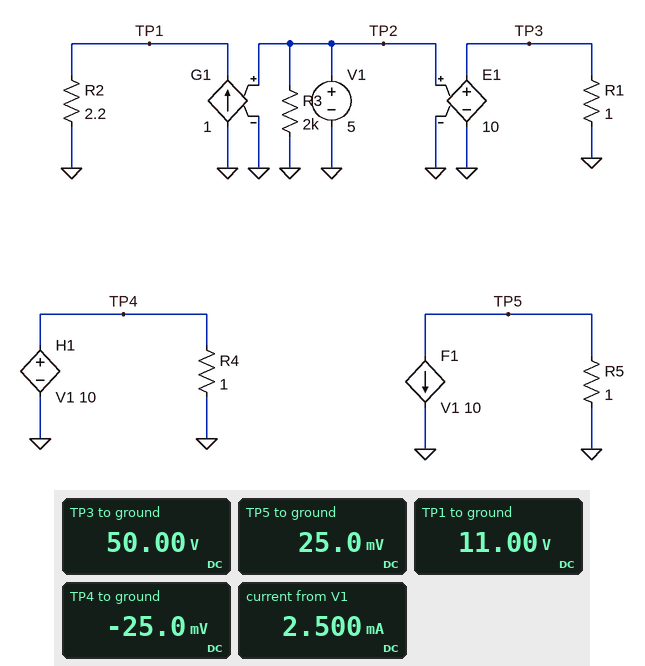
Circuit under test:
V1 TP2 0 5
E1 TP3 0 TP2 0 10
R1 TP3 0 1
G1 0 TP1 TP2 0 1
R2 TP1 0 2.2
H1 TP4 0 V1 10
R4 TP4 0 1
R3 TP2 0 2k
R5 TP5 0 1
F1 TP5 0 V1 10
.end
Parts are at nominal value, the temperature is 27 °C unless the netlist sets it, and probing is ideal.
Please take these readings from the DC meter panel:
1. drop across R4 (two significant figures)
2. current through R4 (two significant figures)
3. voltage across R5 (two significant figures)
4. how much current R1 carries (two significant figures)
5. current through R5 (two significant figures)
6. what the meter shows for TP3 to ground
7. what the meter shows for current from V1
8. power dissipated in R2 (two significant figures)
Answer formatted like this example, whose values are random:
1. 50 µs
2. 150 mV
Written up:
1. 25 mV
2. 25 mA
3. 25 mV
4. 50 A
5. 25 mA
6. 50.00 V
7. 2.500 mA
8. 55 W
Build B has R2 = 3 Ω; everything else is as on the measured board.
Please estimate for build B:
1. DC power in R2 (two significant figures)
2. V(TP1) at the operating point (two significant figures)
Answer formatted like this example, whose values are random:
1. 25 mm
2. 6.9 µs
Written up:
1. 75 W
2. 15 V
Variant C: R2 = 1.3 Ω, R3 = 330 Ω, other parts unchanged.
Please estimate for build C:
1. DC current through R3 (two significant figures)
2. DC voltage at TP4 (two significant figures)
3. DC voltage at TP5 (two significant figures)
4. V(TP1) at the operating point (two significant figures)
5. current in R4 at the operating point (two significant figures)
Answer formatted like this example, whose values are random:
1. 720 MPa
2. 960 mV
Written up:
1. 15 mA
2. -150 mV
3. 150 mV
4. 6.5 V
5. 150 mA
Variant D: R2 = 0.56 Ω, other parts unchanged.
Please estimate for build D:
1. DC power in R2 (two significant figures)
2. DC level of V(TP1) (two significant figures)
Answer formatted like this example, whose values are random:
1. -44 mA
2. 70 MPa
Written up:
1. 14 W
2. 2.8 V
